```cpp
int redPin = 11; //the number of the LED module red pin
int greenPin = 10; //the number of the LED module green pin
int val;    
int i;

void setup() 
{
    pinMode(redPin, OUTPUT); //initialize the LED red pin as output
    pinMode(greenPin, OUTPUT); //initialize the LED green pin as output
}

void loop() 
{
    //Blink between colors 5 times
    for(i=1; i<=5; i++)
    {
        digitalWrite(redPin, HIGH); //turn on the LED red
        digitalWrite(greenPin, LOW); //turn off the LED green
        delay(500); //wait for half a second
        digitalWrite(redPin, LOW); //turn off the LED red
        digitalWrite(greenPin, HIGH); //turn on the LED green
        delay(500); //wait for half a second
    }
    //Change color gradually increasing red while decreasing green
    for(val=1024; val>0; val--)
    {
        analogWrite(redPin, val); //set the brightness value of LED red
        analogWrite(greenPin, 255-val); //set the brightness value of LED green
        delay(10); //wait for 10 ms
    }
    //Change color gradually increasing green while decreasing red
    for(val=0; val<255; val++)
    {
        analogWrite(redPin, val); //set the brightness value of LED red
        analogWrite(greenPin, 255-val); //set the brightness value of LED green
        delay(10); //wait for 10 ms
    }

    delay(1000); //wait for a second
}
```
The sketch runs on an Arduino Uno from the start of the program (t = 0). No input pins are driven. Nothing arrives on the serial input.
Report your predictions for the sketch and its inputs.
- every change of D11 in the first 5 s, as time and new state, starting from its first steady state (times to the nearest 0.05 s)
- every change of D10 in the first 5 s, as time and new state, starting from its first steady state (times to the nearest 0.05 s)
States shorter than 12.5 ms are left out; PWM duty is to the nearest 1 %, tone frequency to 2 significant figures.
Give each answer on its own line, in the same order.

0 s high; 0.5 s low; 1 s high; 1.5 s low; 2 s high; 2.5 s low; 3 s high; 3.5 s low; 4 s high; 4.5 s low
0 s low; 0.5 s high; 1 s low; 1.5 s high; 2 s low; 2.5 s high; 3 s low; 3.5 s high; 4 s low; 4.5 s high
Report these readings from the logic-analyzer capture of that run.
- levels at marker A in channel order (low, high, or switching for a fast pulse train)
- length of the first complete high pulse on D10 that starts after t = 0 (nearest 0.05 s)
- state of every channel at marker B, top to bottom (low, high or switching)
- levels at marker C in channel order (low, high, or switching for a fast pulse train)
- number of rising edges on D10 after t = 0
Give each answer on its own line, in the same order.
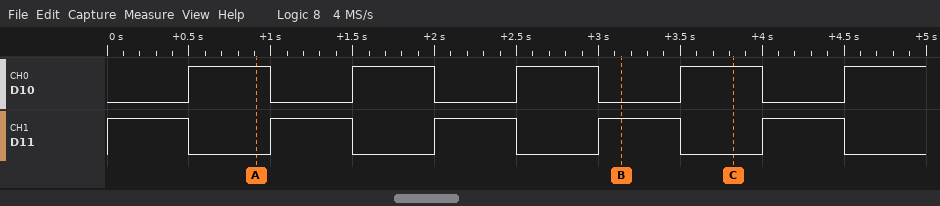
D10 high, D11 low
0.50 s
D10 low, D11 high
D10 high, D11 low
5
